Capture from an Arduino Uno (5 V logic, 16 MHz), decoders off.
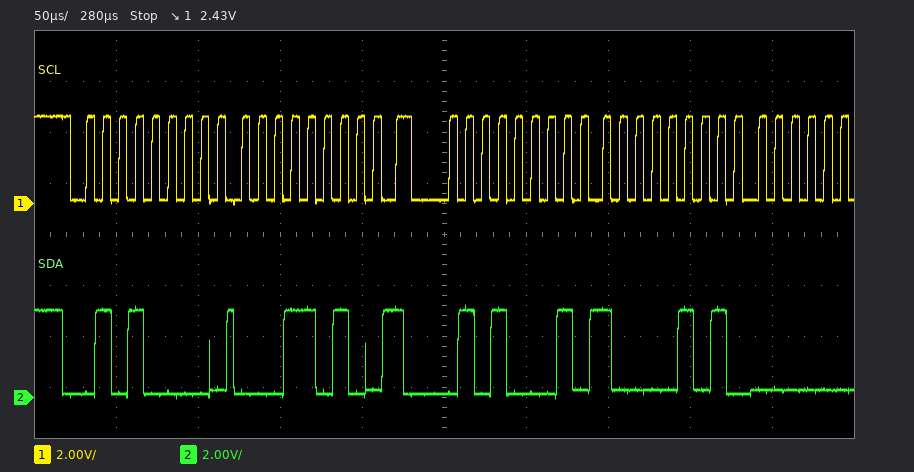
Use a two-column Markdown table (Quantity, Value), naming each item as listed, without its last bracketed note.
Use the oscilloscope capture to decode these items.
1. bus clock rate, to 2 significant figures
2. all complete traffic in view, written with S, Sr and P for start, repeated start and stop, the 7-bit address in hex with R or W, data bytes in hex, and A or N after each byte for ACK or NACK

| Quantity | Value |
|---|---|
| bus clock rate, to 2 significant figures | 100 kHz |
| all complete traffic in view, written with S, Sr and P for start, repeated start and stop, the 7-bit address in hex with R or W, data bytes in hex, and A or N after each byte for ACK or NACK | S 28W A 1A A Sr 28R A 85 A |
